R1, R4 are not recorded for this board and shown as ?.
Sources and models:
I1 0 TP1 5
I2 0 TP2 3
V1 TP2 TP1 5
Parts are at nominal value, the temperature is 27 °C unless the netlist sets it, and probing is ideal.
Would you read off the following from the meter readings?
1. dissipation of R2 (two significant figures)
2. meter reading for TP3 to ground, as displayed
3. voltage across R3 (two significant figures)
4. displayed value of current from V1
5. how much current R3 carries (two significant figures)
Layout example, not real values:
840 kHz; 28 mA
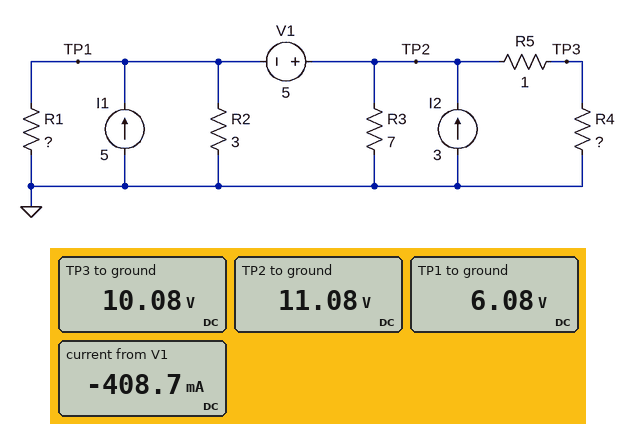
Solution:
12 W; 10.08 V; 11 V; -408.7 mA; 1.6 A
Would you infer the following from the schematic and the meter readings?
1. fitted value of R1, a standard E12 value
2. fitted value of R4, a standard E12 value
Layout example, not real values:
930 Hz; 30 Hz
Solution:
1.8 Ω; 10 Ω
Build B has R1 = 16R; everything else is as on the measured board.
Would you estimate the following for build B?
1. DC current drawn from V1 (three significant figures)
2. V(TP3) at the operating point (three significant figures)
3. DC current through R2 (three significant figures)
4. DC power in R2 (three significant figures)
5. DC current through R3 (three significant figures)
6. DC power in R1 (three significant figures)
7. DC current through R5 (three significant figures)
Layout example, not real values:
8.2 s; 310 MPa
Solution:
705 mA; 14.4 V; 3.62 A; 39.2 W; 2.26 A; 7.36 W; 1.44 A
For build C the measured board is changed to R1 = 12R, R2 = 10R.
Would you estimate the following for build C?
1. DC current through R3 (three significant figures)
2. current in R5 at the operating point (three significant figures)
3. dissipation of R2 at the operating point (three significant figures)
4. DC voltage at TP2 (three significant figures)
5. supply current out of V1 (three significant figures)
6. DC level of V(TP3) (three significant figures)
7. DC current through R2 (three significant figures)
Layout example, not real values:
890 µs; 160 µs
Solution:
3.05 A; 1.94 A; 26.8 W; 21.4 V; 2.00 A; 19.4 V; 1.64 A
